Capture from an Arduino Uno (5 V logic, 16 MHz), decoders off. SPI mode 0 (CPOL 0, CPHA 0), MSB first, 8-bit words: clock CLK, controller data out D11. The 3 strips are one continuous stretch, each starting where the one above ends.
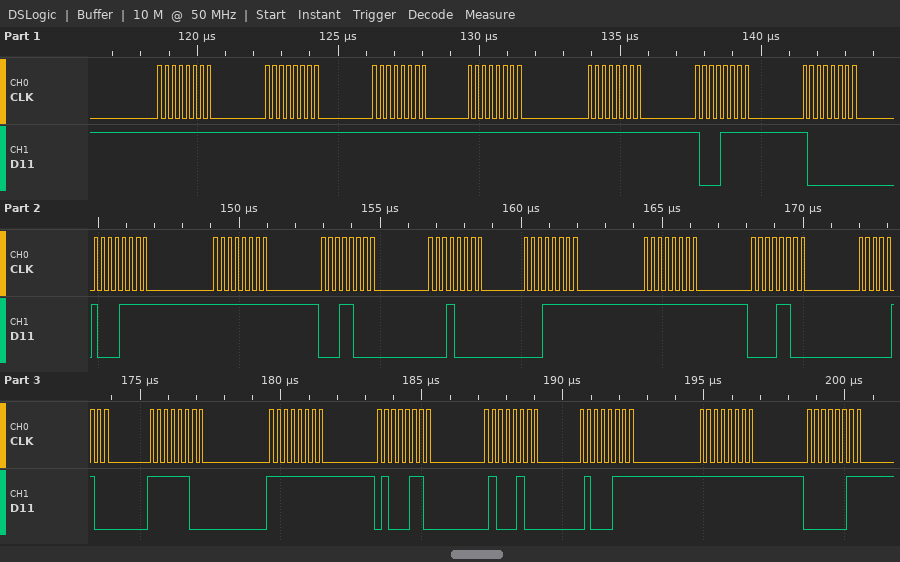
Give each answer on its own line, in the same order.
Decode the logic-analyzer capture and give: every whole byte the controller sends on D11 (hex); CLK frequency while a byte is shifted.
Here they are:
0xFF 0xFF 0xFF 0xFF 0xFF 0x8F 0x80 0x8F 0xFF 0x18 0x10 0x1F 0xFF 0x0C 0x04 0xFC 0xFF 0x46 0x44 0x47 0xFF 0x03
4 MHz
